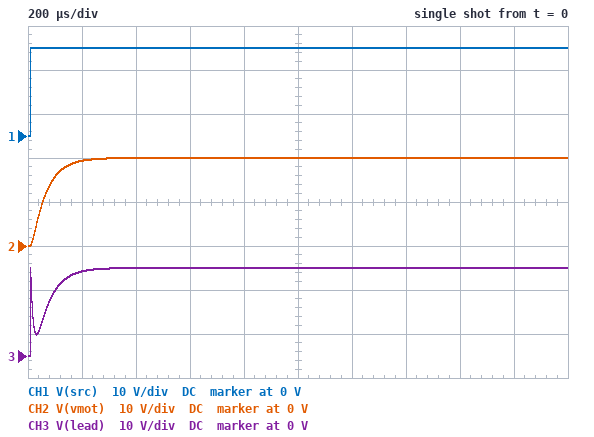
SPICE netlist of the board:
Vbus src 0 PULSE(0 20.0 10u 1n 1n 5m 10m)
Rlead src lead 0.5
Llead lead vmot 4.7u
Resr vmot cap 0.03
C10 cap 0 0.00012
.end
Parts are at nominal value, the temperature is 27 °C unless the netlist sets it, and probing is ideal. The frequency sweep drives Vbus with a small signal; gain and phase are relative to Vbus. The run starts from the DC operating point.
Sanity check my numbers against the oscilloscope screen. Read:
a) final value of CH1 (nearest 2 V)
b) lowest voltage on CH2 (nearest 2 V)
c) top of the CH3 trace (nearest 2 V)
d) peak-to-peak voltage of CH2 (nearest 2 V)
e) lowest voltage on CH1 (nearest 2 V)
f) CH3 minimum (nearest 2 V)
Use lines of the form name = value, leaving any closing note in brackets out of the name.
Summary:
final value of CH1 = 20 V
lowest voltage on CH2 = 0 V
top of the CH3 trace = 20 V
peak-to-peak voltage of CH2 = 20 V
lowest voltage on CH1 = 0 V
CH3 minimum = 0 V
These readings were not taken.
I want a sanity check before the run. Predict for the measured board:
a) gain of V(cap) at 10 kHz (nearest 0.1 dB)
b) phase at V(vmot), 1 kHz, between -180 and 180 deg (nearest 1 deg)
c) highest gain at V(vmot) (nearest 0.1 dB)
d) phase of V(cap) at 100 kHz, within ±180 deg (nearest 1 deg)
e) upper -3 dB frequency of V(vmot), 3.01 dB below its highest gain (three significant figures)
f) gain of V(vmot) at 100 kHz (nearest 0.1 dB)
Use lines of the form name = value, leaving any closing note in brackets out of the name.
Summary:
gain of V(cap) at 10 kHz = -12.4 dB
phase at V(vmot), 1 kHz, between -180 and 180 deg = -21 deg
highest gain at V(vmot) = 0 dB
phase of V(cap) at 100 kHz, within ±180 deg = -170 deg
upper -3 dB frequency of V(vmot), 3.01 dB below its highest gain = 2.91 kHz
gain of V(vmot) at 100 kHz = -39.2 dB
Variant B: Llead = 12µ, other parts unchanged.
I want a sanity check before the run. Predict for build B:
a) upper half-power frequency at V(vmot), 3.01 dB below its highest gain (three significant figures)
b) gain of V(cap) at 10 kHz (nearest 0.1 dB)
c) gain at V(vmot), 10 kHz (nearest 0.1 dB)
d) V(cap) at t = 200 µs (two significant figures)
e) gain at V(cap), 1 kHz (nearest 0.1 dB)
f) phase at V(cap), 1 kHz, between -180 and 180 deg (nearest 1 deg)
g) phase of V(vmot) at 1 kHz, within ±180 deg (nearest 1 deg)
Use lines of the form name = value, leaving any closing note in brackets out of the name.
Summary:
upper half-power frequency at V(vmot), 3.01 dB below its highest gain = 3.46 kHz
gain of V(cap) at 10 kHz = -15.8 dB
gain at V(vmot), 10 kHz = -15.6 dB
V(cap) at t = 200 µs = 20 V
gain at V(cap), 1 kHz = -0.2 dB
phase at V(cap), 1 kHz, between -180 and 180 deg = -23 deg
phase of V(vmot) at 1 kHz, within ±180 deg = -22 deg
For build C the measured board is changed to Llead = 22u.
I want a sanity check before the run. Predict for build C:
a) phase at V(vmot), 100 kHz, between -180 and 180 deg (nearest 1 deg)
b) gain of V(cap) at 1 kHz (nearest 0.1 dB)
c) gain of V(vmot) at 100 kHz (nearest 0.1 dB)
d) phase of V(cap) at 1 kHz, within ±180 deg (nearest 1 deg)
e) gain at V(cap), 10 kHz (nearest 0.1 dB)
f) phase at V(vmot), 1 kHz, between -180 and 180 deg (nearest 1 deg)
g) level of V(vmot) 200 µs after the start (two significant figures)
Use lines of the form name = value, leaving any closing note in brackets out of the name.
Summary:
phase at V(vmot), 100 kHz, between -180 and 180 deg = -112 deg
gain of V(cap) at 1 kHz = 0.2 dB
gain of V(vmot) at 100 kHz = -52.5 dB
phase of V(cap) at 1 kHz, within ±180 deg = -24 deg
gain at V(cap), 10 kHz = -20.2 dB
phase at V(vmot), 1 kHz, between -180 and 180 deg = -23 deg
level of V(vmot) 200 µs after the start = 22 V
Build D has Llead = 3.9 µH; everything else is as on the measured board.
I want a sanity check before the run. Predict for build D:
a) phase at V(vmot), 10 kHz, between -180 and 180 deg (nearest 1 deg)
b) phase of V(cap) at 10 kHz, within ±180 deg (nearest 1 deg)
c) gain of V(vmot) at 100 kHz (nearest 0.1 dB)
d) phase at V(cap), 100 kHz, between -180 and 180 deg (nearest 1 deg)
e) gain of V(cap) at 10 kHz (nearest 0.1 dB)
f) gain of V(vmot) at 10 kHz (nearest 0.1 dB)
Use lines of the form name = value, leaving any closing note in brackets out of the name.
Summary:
phase at V(vmot), 10 kHz, between -180 and 180 deg = -89 deg
phase of V(cap) at 10 kHz, within ±180 deg = -102 deg
gain of V(vmot) at 100 kHz = -37.6 dB
phase at V(cap), 100 kHz, between -180 and 180 deg = -168 deg
gain of V(cap) at 10 kHz = -12.2 dB
gain of V(vmot) at 10 kHz = -12.0 dB
